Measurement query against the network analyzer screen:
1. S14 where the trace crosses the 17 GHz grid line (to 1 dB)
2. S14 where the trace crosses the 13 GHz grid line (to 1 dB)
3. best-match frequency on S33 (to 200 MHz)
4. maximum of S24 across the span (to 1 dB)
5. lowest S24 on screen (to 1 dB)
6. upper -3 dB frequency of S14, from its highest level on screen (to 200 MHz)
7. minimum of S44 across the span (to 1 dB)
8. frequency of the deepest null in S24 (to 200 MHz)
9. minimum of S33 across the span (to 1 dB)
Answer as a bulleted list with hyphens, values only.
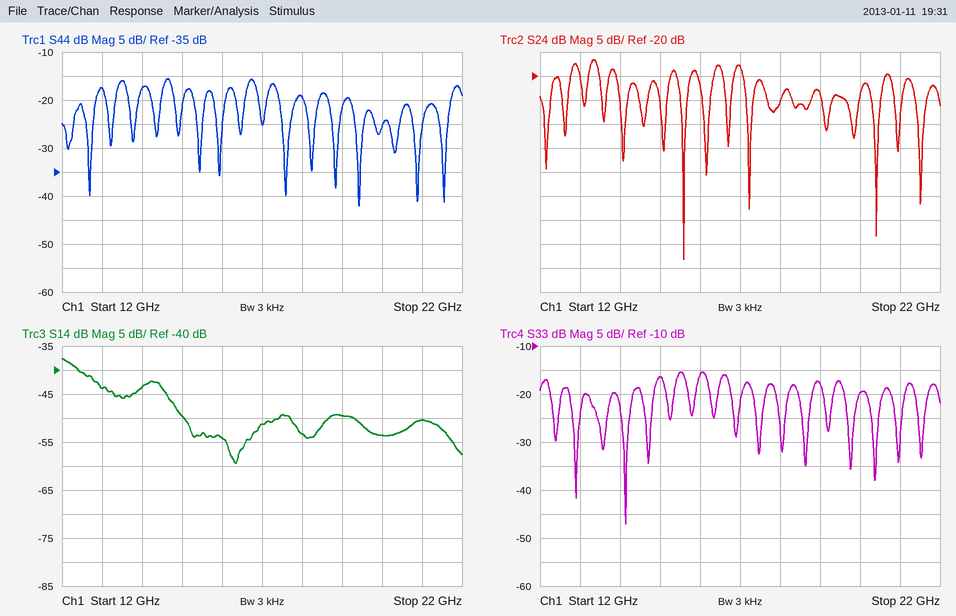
- -51 dB
- -44 dB
- 14.2 GHz
- -17 dB
- -58 dB
- 12.6 GHz
- -42 dB
- 15.6 GHz
- -47 dB
